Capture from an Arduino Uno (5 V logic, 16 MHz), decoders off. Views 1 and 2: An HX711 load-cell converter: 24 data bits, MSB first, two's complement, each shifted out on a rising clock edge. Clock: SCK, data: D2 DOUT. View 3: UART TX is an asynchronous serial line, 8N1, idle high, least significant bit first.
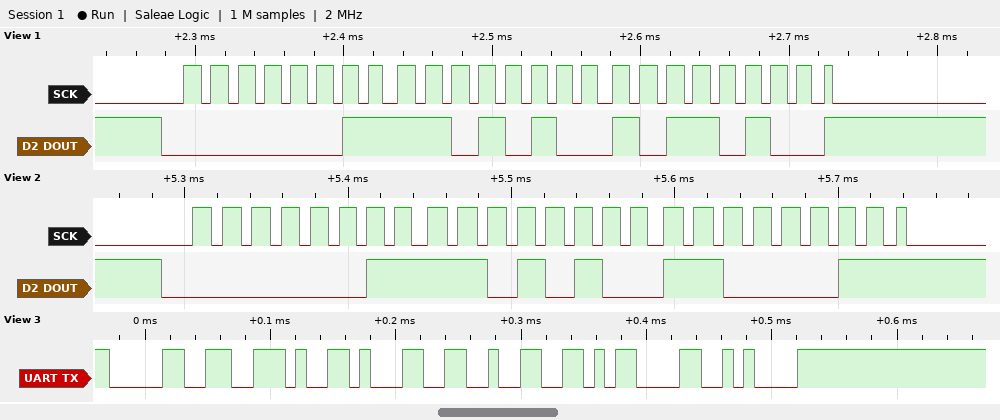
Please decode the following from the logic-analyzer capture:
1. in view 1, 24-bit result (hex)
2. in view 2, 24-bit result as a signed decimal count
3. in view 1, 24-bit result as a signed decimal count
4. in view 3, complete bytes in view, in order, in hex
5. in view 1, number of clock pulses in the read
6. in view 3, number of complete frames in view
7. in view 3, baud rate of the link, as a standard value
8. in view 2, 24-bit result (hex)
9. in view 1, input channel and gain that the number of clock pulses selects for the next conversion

0x03D4B4
251075
251060
0x30 0x2E 0x31 0x32 0x0D 0x0A
25
6
115200 baud
0x03D4C3
channel A, gain 128
